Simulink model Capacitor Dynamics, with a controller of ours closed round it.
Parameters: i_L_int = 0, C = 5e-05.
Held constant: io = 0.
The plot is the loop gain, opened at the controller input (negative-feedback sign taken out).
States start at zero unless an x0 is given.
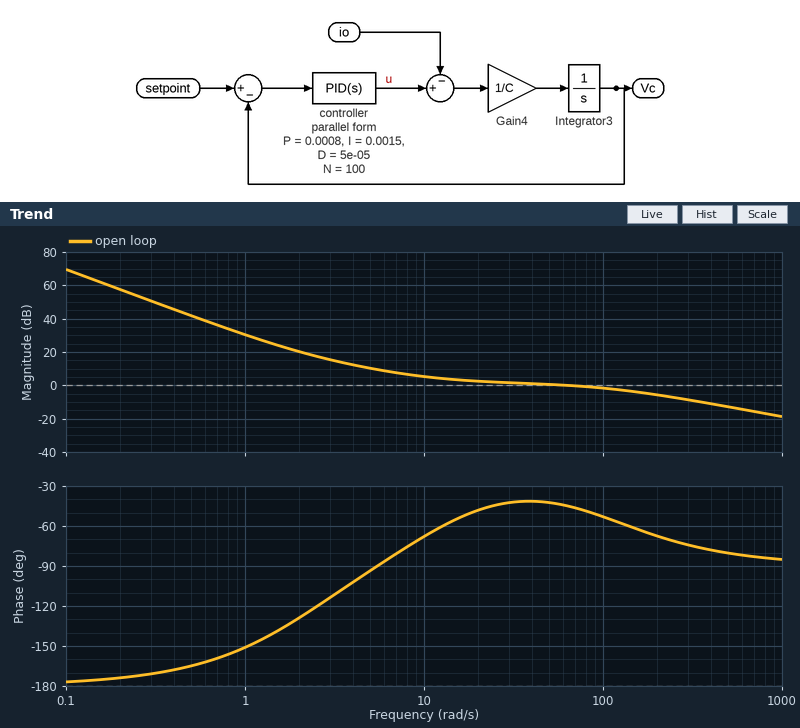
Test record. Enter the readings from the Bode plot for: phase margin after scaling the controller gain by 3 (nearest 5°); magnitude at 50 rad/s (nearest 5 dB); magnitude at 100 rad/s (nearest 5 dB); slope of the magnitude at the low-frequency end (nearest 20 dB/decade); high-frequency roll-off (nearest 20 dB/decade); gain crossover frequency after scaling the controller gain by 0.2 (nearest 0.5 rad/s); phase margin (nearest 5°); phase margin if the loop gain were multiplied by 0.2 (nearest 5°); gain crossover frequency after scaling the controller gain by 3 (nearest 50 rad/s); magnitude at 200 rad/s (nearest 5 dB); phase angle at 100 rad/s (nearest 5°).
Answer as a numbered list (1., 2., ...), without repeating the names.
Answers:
1. 105°
2. 0 dB
3. 0 dB
4. -40 dB/decade
5. -20 dB/decade
6. 3.5 rad/s
7. 135°
8. 70°
9. 350 rad/s
10. -5 dB
11. -55°
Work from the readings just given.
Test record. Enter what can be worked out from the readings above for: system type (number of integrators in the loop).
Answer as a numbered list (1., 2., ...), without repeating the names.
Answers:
1. 2
